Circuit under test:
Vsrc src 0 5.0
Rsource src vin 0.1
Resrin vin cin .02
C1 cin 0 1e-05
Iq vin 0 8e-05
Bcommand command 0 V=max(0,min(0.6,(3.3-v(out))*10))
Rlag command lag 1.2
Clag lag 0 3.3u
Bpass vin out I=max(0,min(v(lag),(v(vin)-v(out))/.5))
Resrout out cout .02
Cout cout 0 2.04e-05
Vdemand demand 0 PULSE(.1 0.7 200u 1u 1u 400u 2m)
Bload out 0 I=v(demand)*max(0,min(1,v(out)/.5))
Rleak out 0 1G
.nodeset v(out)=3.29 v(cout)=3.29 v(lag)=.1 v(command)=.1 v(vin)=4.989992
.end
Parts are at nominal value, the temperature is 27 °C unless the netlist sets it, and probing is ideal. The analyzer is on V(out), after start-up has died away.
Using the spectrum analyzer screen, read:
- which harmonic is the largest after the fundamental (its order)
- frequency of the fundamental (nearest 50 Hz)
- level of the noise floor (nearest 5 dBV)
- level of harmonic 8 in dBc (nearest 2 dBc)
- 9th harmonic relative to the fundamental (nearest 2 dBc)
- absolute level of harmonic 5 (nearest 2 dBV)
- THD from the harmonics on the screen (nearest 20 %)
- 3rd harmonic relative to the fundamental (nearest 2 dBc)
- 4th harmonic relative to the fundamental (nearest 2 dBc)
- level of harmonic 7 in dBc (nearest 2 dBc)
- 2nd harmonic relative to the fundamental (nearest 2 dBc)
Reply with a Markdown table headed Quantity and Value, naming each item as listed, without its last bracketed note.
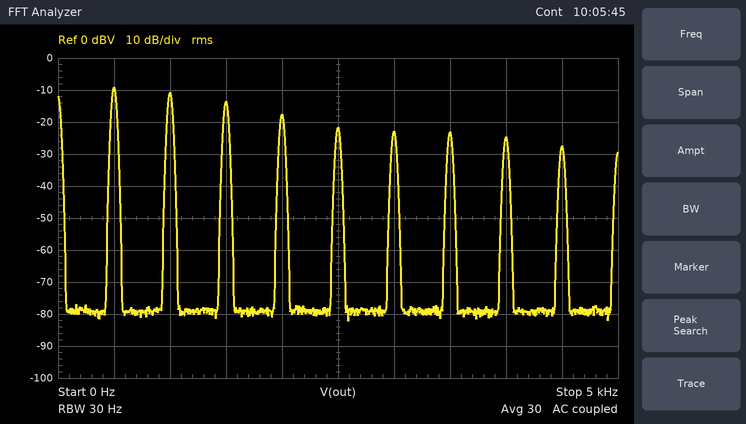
| Quantity | Value |
|---|---|
| which harmonic is the largest after the fundamental | 2 |
| frequency of the fundamental | 500 Hz |
| level of the noise floor | -80 dBV |
| level of harmonic 8 in dBc | -16 dBc |
| 9th harmonic relative to the fundamental | -18 dBc |
| absolute level of harmonic 5 | -22 dBV |
| THD from the harmonics on the screen | 120 % |
| 3rd harmonic relative to the fundamental | -4 dBc |
| 4th harmonic relative to the fundamental | -8 dBc |
| level of harmonic 7 in dBc | -14 dBc |
| 2nd harmonic relative to the fundamental | -2 dBc |
